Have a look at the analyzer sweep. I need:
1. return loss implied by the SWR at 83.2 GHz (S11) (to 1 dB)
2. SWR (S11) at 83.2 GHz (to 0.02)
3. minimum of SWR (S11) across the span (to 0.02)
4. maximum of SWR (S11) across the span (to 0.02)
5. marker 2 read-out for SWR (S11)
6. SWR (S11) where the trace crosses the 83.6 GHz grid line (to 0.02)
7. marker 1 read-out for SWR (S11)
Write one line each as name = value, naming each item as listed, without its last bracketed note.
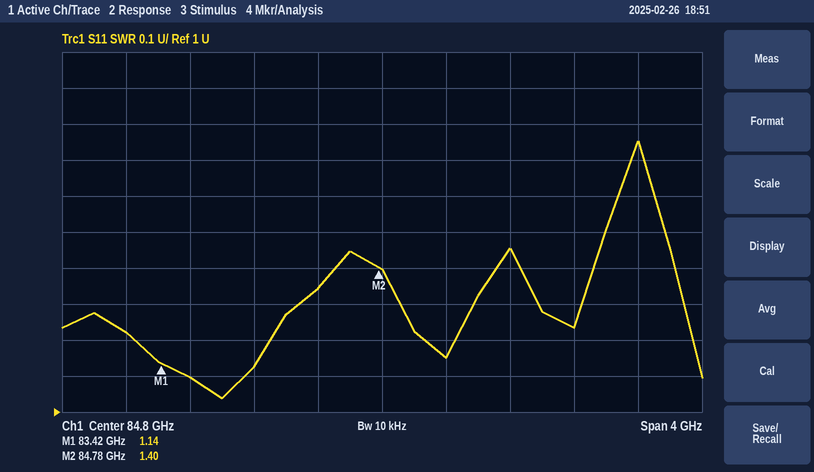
return loss implied by the SWR at 83.2 GHz (S11) = 20 dB
SWR (S11) at 83.2 GHz = 1.22
minimum of SWR (S11) across the span = 1.04
maximum of SWR (S11) across the span = 1.76
marker 2 read-out for SWR = 1.40
SWR (S11) where the trace crosses the 83.6 GHz grid line = 1.10
marker 1 read-out for SWR = 1.14
